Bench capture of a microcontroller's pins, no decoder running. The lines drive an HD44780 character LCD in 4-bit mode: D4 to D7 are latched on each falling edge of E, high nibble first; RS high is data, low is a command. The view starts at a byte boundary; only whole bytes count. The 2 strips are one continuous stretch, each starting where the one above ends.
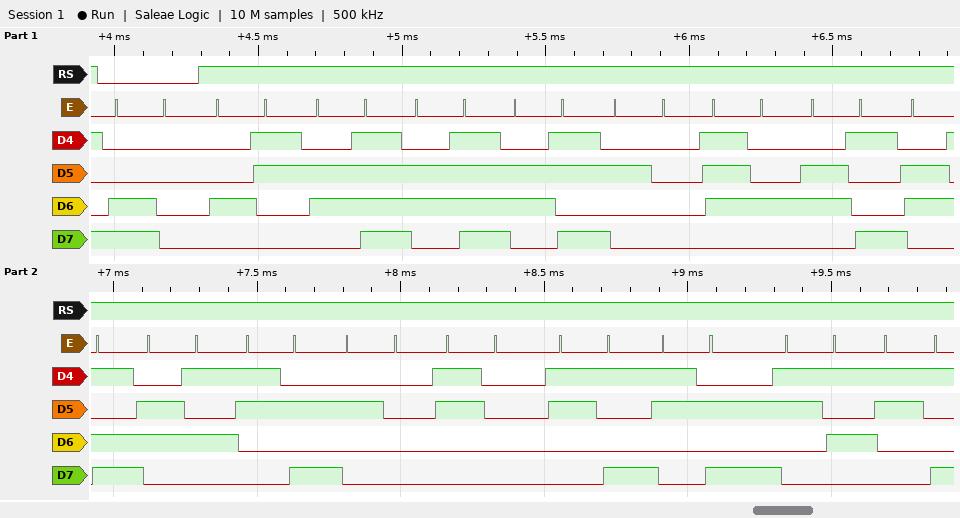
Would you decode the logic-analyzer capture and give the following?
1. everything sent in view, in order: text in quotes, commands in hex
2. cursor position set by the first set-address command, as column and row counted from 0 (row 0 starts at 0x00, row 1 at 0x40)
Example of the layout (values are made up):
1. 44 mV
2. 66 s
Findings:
1. 0xC0 "Cook time: 09:59"
2. column 0, row 1
